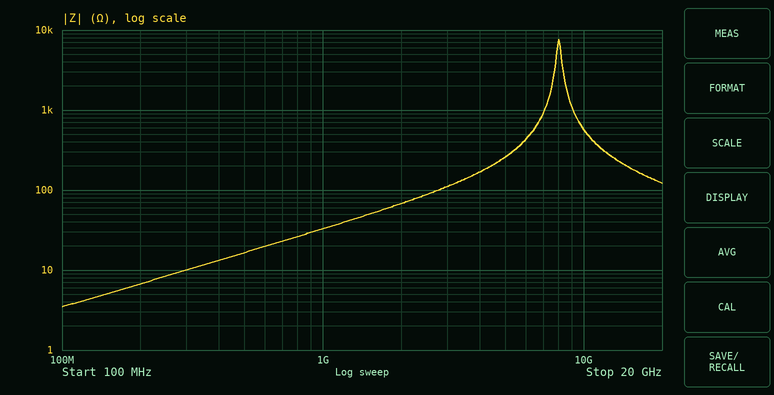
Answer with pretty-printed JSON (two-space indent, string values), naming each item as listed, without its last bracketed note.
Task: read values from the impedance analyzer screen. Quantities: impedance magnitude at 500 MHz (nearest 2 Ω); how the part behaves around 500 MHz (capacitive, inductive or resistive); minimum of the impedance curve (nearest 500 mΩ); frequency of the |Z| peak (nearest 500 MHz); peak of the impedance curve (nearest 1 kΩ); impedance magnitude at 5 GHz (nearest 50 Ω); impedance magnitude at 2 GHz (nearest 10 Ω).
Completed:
{
  "impedance magnitude at 500 MHz": "16 Ω",
  "how the part behaves around 500 MHz": "inductive",
  "minimum of the impedance curve": "3.5 Ω",
  "frequency of the |Z| peak": "8.0 GHz",
  "peak of the impedance curve": "8 kΩ",
  "impedance magnitude at 5 GHz": "250 Ω",
  "impedance magnitude at 2 GHz": "70 Ω"
}
